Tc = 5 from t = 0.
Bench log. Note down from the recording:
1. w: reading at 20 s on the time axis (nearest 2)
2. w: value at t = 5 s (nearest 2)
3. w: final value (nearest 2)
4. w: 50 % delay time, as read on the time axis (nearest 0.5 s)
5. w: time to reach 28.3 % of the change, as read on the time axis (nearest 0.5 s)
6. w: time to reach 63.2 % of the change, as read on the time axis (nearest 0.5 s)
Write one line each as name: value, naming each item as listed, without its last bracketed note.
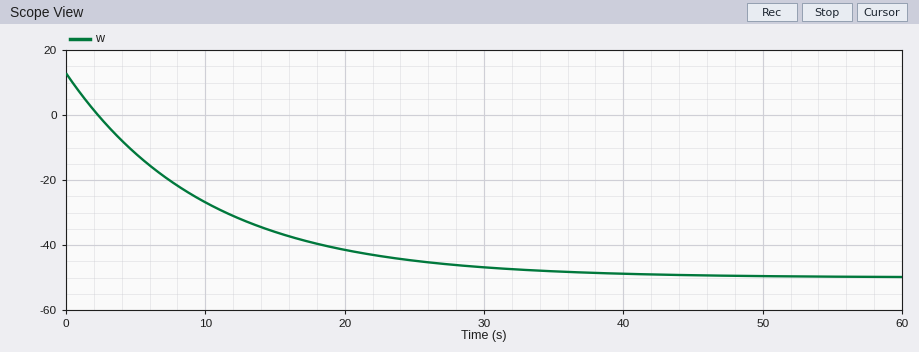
w: reading at 20 s on the time axis: -42
w: value at t = 5 s: -12
w: final value: -50
w: 50 % delay time, as read on the time axis: 7.0 s
w: time to reach 28.3 % of the change, as read on the time axis: 3.5 s
w: time to reach 63.2 % of the change, as read on the time axis: 10.0 s
